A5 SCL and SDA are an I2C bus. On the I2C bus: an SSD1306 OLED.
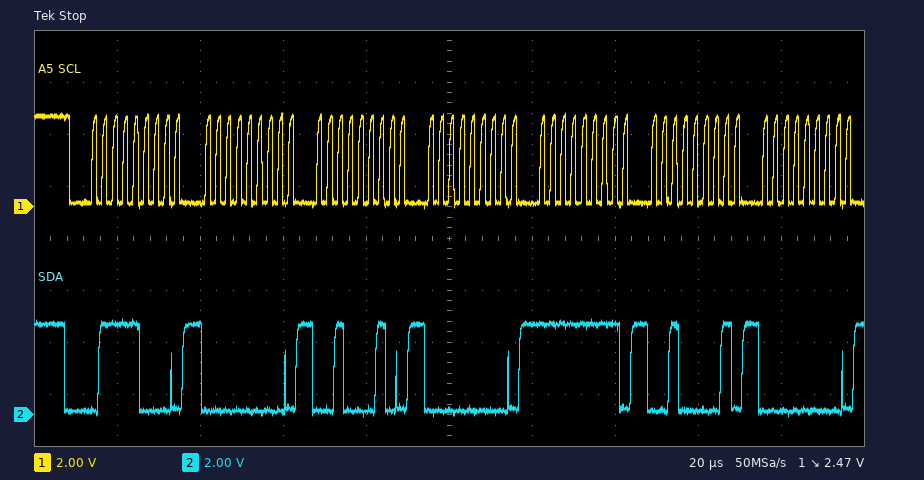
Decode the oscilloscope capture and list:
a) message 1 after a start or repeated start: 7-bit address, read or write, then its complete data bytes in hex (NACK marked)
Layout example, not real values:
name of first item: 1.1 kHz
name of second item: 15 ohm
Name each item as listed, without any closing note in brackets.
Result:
message 1 after a start or repeated start: 7-bit address, read or write, then its complete data bytes in hex: 0x3C write: 00 22 00 FF 21 00
